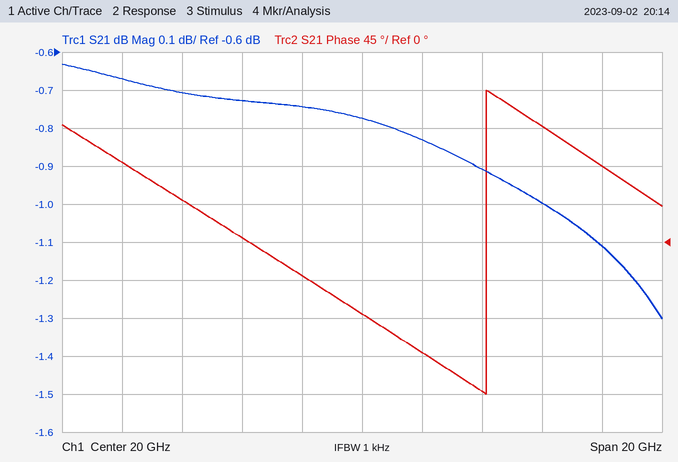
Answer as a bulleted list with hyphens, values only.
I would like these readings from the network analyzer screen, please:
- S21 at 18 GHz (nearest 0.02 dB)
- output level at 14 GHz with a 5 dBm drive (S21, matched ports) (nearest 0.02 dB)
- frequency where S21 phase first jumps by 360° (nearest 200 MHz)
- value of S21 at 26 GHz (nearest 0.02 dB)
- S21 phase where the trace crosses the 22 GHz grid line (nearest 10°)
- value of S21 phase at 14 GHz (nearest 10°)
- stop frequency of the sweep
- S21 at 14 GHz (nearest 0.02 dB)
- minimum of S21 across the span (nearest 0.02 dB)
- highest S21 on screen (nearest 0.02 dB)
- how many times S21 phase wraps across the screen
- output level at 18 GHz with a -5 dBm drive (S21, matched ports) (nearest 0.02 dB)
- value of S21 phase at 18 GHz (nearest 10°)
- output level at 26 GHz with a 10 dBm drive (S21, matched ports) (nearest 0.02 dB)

- -0.74 dB
- 4.30 dBm
- 24.2 GHz
- -1.00 dB
- -130°
- 50°
- 30 GHz
- -0.70 dB
- -1.30 dB
- -0.64 dB
- 1
- -5.74 dBm
- -40°
- 9.00 dBm
